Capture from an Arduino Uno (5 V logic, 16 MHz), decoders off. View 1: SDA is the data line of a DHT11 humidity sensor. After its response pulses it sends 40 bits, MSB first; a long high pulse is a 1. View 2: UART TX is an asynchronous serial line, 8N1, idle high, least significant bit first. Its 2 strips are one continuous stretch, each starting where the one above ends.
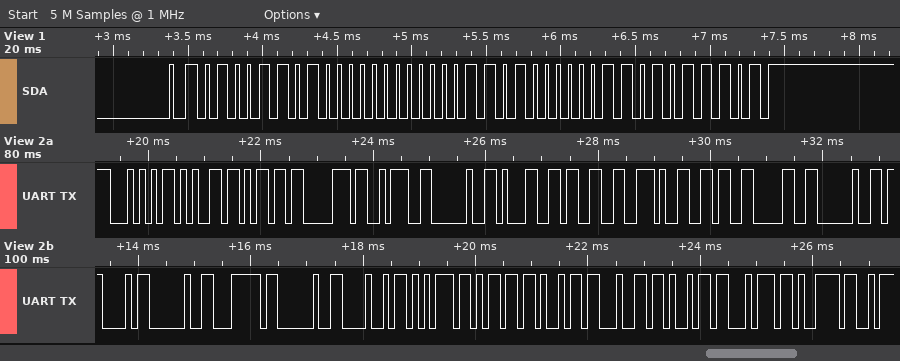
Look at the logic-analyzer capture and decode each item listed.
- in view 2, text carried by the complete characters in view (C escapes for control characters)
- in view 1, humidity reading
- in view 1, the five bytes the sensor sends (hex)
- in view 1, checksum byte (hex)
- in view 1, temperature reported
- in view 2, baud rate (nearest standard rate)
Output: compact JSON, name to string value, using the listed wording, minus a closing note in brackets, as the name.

{"in view 2, text carried by the complete characters in view": "\"Temp: 13.60 C | Humidity\"", "in view 1, humidity reading": "77 %", "in view 1, the five bytes the sensor sends": "4D 00 0D 03 5D", "in view 1, checksum byte": "0x5D", "in view 1, temperature reported": "13.3 °C", "in view 2, baud rate": "9600 baud"}
